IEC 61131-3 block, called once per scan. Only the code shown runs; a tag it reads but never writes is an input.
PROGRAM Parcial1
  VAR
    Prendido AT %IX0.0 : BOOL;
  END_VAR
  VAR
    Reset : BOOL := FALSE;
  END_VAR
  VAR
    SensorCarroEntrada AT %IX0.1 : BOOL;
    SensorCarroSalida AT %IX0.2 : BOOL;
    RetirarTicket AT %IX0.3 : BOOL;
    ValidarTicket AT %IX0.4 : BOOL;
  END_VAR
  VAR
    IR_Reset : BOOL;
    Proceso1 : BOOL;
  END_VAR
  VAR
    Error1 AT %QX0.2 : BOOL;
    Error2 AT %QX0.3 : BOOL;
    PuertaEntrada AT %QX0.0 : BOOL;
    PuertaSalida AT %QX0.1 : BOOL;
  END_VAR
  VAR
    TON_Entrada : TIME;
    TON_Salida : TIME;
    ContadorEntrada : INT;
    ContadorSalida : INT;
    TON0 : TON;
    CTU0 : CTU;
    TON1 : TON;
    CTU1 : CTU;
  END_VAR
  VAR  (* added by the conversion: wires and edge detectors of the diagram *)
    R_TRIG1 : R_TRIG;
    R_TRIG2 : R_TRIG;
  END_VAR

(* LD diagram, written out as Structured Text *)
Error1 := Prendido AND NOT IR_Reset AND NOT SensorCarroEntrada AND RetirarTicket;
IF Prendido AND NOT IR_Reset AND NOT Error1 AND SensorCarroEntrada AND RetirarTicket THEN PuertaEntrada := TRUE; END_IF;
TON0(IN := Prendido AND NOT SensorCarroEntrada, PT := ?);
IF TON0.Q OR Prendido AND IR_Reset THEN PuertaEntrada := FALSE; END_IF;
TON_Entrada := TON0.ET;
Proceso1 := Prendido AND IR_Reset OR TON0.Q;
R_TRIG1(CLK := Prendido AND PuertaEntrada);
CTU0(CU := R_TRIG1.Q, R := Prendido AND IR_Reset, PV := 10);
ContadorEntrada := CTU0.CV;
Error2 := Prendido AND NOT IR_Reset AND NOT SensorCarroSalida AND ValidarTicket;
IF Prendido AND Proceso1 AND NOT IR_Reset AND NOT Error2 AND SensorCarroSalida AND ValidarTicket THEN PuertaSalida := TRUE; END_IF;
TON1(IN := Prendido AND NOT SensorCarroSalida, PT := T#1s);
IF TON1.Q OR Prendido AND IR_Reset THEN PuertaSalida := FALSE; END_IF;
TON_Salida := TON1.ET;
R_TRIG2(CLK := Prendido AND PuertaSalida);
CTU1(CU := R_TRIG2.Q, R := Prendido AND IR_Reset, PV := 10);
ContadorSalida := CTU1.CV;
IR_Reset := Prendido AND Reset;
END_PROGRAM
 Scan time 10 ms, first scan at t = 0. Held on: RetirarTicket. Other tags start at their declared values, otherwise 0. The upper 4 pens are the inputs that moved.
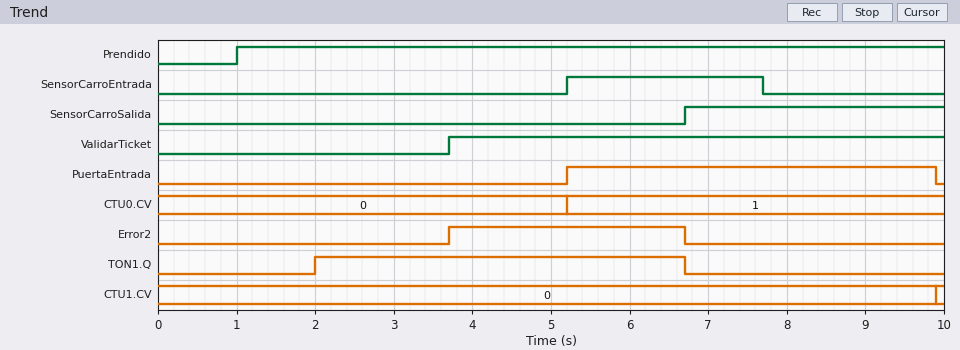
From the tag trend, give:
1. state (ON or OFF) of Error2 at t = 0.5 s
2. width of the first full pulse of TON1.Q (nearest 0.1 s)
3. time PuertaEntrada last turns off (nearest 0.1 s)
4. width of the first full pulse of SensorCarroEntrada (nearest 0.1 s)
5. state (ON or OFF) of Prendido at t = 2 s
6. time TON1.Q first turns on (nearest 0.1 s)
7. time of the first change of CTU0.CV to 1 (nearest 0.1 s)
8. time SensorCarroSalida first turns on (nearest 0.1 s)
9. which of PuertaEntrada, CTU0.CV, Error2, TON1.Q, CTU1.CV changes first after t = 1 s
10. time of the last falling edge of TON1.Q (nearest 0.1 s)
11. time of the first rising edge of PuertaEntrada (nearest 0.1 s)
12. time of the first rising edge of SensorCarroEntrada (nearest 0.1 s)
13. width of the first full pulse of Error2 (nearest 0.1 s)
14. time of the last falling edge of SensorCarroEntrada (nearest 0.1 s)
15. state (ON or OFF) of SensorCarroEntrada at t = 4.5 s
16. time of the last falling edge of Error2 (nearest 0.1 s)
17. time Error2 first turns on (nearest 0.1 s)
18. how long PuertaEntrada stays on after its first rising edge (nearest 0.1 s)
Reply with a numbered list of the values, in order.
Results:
1. OFF
2. 4.7 s
3. 9.9 s
4. 2.5 s
5. ON
6. 2.0 s
7. 5.2 s
8. 6.7 s
9. TON1.Q
10. 6.7 s
11. 5.2 s
12. 5.2 s
13. 3.0 s
14. 7.7 s
15. OFF
16. 6.7 s
17. 3.7 s
18. 4.7 s
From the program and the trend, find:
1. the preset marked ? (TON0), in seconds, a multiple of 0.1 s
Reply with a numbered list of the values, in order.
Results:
1. 2.2 s
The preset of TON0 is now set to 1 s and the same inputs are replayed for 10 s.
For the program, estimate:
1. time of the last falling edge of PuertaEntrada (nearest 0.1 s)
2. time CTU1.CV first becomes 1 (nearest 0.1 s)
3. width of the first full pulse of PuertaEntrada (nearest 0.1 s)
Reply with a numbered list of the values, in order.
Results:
1. 8.7 s
2. 8.7 s
3. 3.5 s
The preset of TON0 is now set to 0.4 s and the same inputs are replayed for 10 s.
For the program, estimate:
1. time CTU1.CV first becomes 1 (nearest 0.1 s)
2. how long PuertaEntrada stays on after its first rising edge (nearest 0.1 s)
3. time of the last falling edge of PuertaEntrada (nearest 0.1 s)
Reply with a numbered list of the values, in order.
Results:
1. 8.1 s
2. 2.9 s
3. 8.1 s
